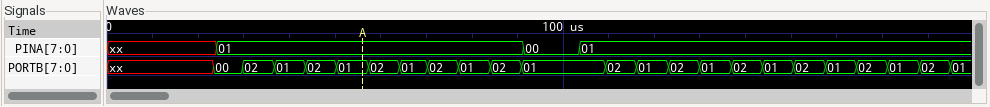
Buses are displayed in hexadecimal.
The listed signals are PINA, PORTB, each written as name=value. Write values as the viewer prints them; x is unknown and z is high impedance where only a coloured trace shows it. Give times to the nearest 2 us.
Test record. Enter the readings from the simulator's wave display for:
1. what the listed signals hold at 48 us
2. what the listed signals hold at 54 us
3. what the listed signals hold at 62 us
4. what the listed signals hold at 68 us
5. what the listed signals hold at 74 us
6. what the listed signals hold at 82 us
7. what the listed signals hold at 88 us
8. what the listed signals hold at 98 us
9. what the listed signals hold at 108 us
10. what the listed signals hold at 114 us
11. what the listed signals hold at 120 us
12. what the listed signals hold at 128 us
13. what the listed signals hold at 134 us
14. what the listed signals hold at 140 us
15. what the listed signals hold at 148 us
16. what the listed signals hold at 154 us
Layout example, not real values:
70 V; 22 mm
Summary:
PINA=01, PORTB=02; PINA=01, PORTB=01; PINA=01, PORTB=02; PINA=01, PORTB=01; PINA=01, PORTB=02; PINA=01, PORTB=01; PINA=01, PORTB=02; PINA=00, PORTB=01; PINA=01, PORTB=01; PINA=01, PORTB=02; PINA=01, PORTB=01; PINA=01, PORTB=02; PINA=01, PORTB=01; PINA=01, PORTB=02; PINA=01, PORTB=01; PINA=01, PORTB=02
